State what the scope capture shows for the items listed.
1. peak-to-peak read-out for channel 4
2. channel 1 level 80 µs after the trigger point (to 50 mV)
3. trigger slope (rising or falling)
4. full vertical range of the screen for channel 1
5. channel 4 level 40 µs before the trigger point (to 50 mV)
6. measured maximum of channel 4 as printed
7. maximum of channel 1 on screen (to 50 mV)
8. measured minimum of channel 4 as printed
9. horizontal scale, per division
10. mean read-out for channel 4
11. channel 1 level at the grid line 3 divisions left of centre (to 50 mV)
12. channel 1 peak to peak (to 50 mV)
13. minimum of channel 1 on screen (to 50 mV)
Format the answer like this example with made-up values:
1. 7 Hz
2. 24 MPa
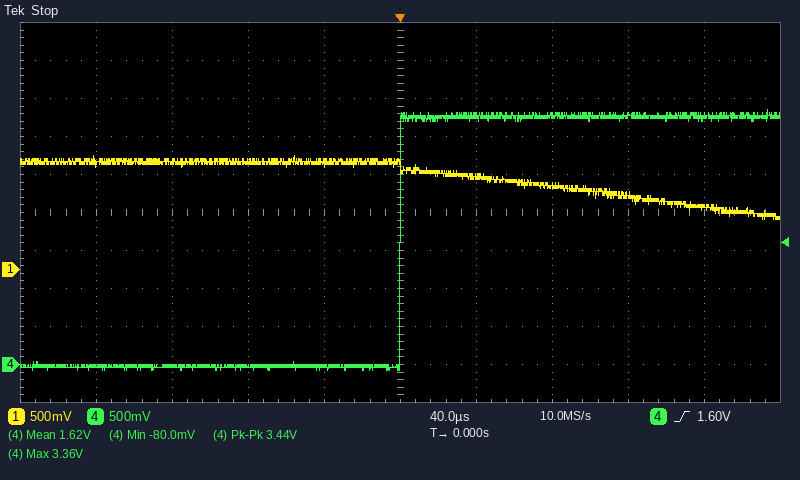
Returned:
1. 3.44 V
2. 1.10 V
3. rising
4. 5 V
5. -50 mV
6. 3.36 V
7. 1.50 V
8. -80.0 mV
9. 40 µs
10. 1.62 V
11. 1.40 V
12. 850 mV
13. 650 mV
